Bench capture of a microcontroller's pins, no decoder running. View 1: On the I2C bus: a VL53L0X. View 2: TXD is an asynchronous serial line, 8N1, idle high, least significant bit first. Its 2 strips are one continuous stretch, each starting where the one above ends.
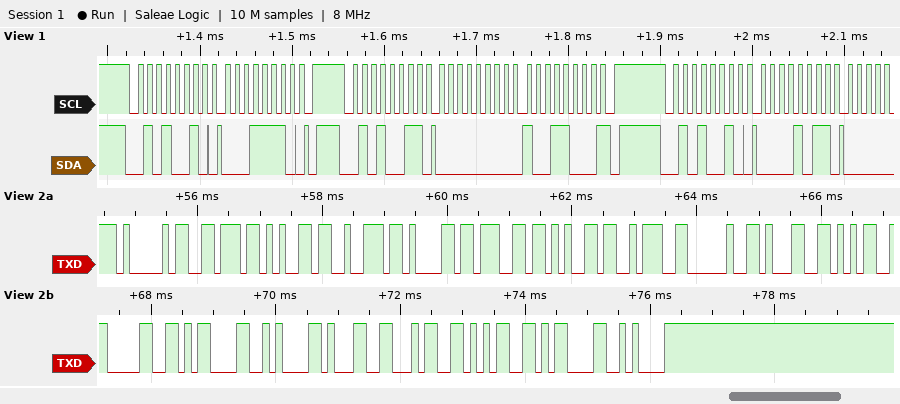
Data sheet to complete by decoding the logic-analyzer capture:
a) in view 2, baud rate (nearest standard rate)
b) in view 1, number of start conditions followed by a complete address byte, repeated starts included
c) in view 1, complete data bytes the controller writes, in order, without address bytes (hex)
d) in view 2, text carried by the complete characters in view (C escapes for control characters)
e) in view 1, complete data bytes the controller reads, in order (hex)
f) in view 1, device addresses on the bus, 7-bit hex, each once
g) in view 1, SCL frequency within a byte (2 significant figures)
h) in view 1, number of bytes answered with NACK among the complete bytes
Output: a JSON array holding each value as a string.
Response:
["9600 baud", "3", "1E 0B", "\"Average: 150\\r\\n145\\r\\n\"", "00 98", "0x29", "100 kHz", "1"]
